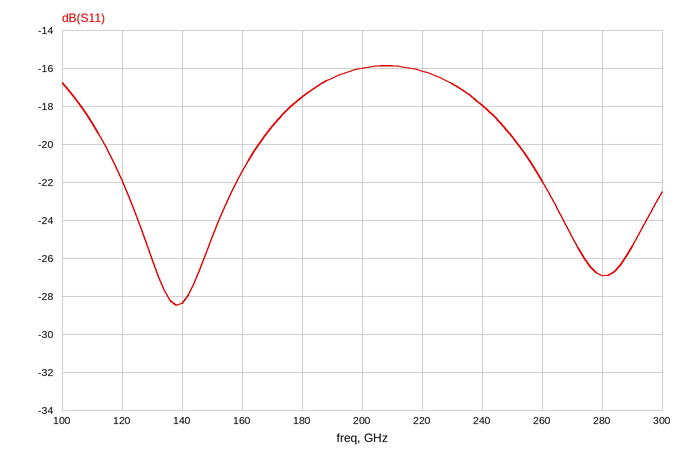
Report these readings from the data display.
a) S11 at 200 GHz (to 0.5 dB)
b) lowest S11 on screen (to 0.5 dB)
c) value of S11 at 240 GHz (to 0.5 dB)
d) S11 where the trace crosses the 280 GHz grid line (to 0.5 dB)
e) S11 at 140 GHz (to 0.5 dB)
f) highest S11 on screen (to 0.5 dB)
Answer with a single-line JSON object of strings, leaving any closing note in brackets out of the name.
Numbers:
{"S11 at 200 GHz": "-16.0 dB", "lowest S11 on screen": "-28.5 dB", "value of S11 at 240 GHz": "-18.0 dB", "S11 where the trace crosses the 280 GHz grid line": "-27.0 dB", "S11 at 140 GHz": "-28.5 dB", "highest S11 on screen": "-16.0 dB"}
